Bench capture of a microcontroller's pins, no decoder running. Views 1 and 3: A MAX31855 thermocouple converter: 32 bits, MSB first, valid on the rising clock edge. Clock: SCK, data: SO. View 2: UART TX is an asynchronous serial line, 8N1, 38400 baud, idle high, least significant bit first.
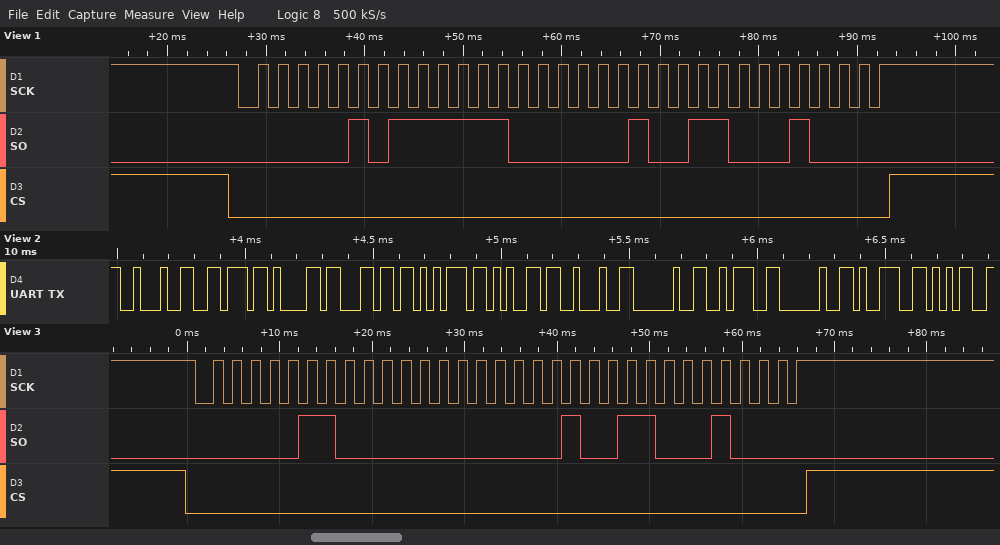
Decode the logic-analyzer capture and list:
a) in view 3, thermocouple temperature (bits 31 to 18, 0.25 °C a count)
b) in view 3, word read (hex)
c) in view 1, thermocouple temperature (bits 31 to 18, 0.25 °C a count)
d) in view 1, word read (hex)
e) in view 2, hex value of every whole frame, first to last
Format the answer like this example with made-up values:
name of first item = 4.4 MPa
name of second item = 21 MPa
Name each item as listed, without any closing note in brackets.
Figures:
in view 3, thermocouple temperature = 96.00 °C
in view 3, word read = 0x06001310
in view 1, thermocouple temperature = 95.50 °C
in view 1, word read = 0x05F81310
in view 2, hex value of every whole frame, first to last = 22 76 61 6C 75 65 22 20 3A 20 39 35
